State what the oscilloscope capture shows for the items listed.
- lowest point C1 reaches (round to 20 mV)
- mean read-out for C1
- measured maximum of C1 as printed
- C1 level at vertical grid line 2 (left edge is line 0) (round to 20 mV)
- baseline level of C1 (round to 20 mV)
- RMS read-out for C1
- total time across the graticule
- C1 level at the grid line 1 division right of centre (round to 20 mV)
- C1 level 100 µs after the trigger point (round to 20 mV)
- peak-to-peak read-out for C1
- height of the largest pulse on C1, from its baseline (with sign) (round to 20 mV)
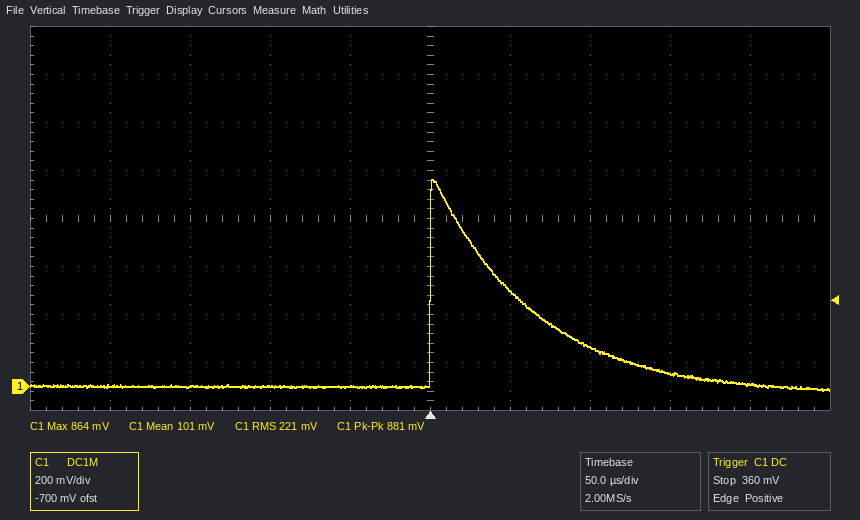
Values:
-20 mV
101 mV
864 mV
0 mV
0 mV
221 mV
500 µs
400 mV
160 mV
881 mV
+860 mV
